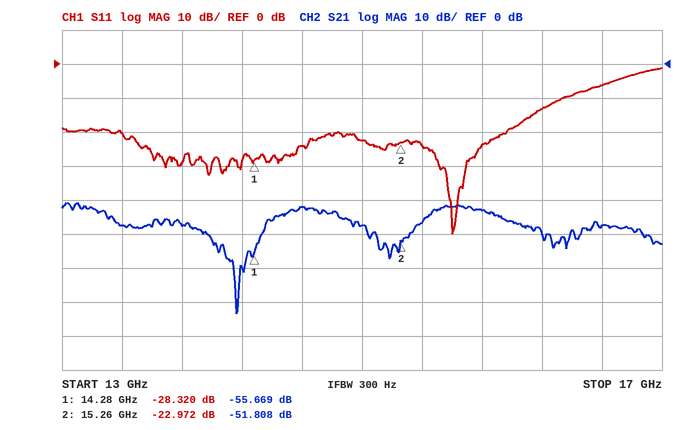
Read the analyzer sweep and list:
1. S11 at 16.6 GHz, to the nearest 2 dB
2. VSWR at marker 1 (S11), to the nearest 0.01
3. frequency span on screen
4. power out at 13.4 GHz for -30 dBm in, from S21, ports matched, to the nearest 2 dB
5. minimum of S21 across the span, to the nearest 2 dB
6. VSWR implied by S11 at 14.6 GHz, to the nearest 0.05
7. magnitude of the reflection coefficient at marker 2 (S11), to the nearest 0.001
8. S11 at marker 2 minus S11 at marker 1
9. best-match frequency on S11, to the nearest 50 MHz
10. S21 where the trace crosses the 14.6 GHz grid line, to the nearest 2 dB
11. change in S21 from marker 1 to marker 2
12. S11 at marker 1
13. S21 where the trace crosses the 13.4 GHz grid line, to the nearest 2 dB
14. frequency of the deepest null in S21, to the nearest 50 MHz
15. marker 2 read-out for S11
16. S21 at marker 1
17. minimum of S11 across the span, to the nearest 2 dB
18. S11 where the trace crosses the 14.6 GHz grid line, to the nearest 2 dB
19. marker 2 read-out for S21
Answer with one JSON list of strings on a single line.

["-6 dB", "1.08", "4 GHz", "-78 dBm", "-74 dB", "1.15", "0.071", "5.348 dB", "15.60 GHz", "-42 dB", "3.861 dB", "-28.320 dB", "-48 dB", "14.15 GHz", "-22.972 dB", "-55.669 dB", "-50 dB", "-24 dB", "-51.808 dB"]
